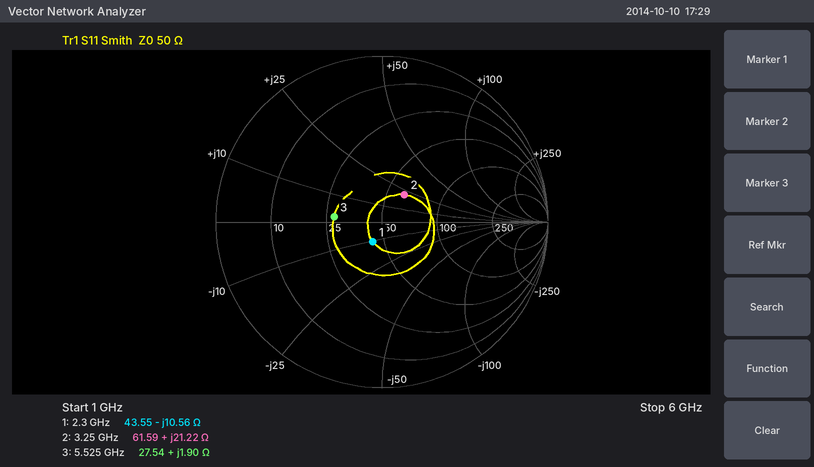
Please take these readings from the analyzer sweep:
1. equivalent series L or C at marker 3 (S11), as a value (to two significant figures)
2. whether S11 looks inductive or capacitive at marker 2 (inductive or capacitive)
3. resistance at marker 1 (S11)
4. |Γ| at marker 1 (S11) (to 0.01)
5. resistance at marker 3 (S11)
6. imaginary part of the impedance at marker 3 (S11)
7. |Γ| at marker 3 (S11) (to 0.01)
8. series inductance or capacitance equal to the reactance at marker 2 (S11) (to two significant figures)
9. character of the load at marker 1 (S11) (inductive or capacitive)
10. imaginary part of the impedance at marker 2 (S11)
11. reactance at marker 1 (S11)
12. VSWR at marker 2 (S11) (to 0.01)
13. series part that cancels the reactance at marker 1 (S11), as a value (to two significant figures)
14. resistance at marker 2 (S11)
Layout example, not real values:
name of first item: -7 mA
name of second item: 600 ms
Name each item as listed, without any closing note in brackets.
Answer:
equivalent series L or C at marker 3 (S11), as a value: 55 pH
whether S11 looks inductive or capacitive at marker 2: inductive
resistance at marker 1: 43.55 Ω
|Γ| at marker 1 (S11): 0.13
resistance at marker 3: 27.54 Ω
imaginary part of the impedance at marker 3: +1.90 Ω
|Γ| at marker 3 (S11): 0.29
series inductance or capacitance equal to the reactance at marker 2 (S11): 1.0 nH
character of the load at marker 1 (S11): capacitive
imaginary part of the impedance at marker 2: +21.22 Ω
reactance at marker 1: -10.56 Ω
VSWR at marker 2 (S11): 1.54
series part that cancels the reactance at marker 1 (S11), as a value: 730 pH
resistance at marker 2: 61.59 Ω
